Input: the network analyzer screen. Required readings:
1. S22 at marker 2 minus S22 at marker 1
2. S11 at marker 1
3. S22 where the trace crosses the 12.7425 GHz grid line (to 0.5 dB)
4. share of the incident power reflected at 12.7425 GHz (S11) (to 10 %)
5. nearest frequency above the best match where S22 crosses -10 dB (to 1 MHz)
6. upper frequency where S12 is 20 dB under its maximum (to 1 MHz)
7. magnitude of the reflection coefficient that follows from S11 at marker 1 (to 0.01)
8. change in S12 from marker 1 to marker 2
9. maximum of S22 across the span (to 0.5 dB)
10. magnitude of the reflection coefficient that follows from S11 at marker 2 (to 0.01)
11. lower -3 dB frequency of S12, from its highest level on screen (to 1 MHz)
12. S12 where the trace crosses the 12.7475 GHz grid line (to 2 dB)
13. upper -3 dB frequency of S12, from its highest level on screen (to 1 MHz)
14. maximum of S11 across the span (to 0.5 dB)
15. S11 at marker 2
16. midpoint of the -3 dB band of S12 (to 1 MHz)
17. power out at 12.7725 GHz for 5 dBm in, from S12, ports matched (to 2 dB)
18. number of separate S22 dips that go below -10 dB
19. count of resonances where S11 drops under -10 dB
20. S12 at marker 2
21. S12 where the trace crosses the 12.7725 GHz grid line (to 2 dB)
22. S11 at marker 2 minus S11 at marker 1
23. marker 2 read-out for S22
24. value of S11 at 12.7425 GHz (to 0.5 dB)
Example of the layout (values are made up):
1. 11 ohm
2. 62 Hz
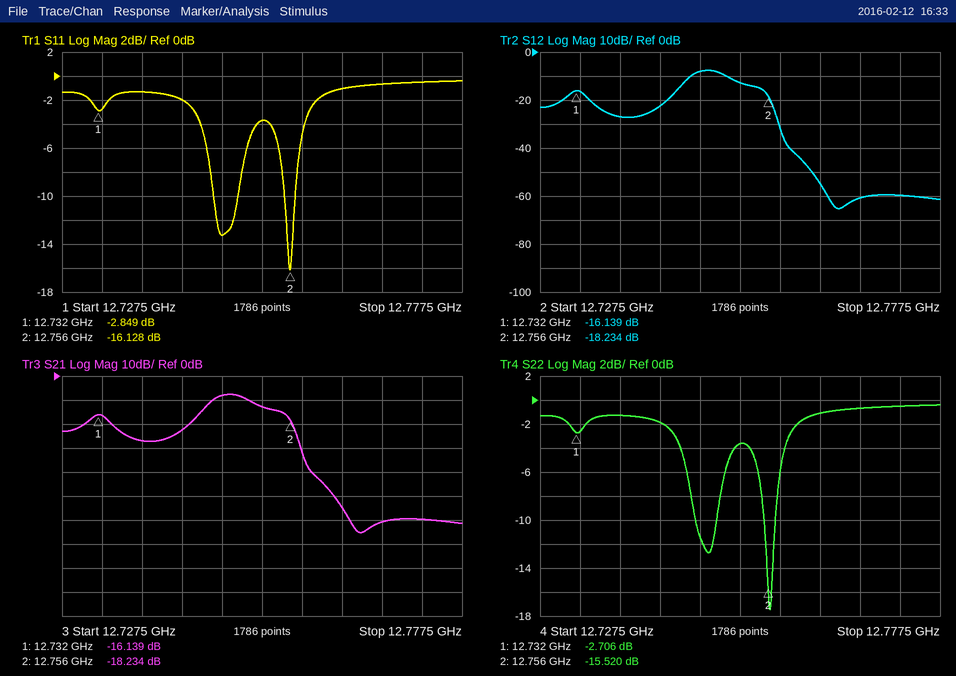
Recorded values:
1. -12.814 dB
2. -2.849 dB
3. -2.0 dB
4. 60 %
5. 12.757 GHz
6. 12.757 GHz
7. 0.72
8. -2.095 dB
9. -0.5 dB
10. 0.16
11. 12.746 GHz
12. -8 dB
13. 12.751 GHz
14. -0.5 dB
15. -16.128 dB
16. 12.749 GHz
17. -54 dBm
18. 2
19. 2
20. -18.234 dB
21. -60 dB
22. -13.279 dB
23. -15.520 dB
24. -2.0 dB
